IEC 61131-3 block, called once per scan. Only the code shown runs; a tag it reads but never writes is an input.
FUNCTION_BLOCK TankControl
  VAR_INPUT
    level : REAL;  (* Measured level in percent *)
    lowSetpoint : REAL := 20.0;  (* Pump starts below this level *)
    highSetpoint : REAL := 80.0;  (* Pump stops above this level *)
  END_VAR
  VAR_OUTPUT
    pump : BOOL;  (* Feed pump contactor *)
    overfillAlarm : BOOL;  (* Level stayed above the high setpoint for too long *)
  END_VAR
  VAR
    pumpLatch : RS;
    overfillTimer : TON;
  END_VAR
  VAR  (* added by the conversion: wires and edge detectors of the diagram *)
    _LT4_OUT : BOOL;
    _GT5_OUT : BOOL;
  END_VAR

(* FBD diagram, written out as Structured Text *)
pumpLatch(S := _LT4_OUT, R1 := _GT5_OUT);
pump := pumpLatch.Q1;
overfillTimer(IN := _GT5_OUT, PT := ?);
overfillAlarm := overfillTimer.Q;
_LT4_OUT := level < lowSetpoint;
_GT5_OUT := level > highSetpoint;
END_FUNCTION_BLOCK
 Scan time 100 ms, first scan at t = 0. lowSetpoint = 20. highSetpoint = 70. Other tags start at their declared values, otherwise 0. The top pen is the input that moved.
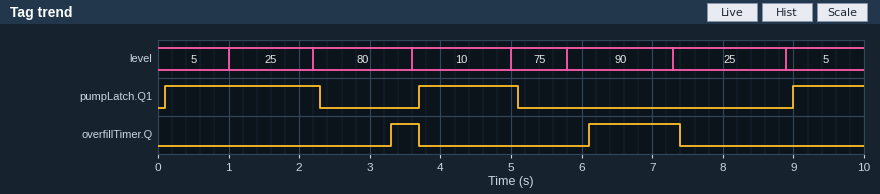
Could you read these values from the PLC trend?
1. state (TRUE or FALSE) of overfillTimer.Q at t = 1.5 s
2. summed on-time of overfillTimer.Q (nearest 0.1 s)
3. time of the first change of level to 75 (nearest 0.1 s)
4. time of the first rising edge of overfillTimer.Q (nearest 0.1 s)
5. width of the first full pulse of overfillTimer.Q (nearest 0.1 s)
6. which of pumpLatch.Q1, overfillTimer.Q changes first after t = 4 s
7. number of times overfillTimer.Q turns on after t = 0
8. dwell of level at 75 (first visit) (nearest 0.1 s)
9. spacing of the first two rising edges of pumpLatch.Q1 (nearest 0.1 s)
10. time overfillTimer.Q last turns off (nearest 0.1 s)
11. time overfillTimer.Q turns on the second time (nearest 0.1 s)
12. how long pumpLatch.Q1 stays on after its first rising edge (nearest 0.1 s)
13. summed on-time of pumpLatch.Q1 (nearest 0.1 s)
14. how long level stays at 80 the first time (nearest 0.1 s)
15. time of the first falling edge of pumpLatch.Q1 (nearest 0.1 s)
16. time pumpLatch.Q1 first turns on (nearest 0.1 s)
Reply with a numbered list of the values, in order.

1. FALSE
2. 1.7 s
3. 5.0 s
4. 3.3 s
5. 0.4 s
6. pumpLatch.Q1
7. 2
8. 0.8 s
9. 3.6 s
10. 7.4 s
11. 6.1 s
12. 2.2 s
13. 4.6 s
14. 1.4 s
15. 2.3 s
16. 0.1 s
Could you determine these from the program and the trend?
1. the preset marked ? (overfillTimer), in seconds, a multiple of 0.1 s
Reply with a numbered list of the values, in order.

1. 1.0 s
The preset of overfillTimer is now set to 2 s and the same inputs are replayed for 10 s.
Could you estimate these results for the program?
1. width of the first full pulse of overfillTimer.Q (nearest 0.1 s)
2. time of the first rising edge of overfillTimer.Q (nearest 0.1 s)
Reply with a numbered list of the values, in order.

1. 0.3 s
2. 7.1 s
